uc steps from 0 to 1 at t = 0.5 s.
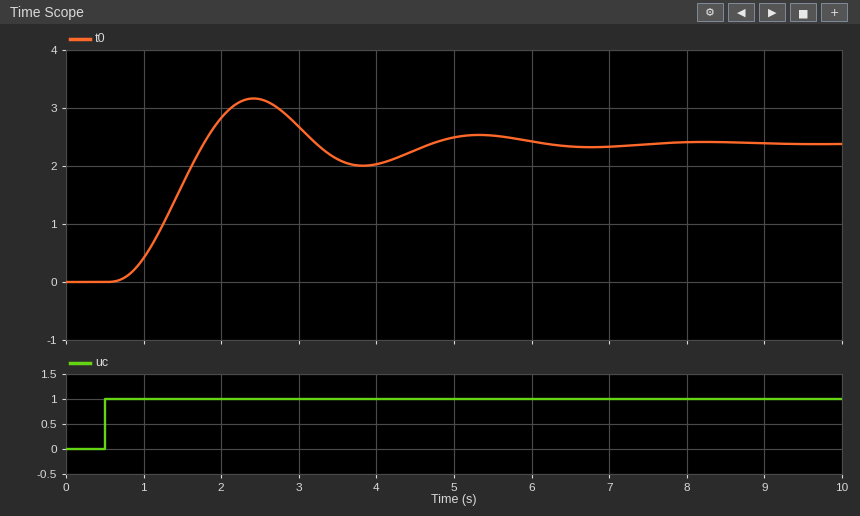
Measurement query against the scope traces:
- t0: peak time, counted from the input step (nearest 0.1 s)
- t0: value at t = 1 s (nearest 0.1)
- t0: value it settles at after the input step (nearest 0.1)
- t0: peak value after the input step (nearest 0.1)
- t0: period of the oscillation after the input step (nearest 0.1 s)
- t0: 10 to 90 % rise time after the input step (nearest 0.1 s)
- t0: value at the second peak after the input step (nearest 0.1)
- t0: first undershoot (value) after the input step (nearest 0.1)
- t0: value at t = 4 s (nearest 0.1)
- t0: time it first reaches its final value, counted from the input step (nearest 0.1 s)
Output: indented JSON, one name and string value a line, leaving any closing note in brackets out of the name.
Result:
{
  "t0: peak time, counted from the input step": "1.9 s",
  "t0: value at t = 1 s": "0.4",
  "t0: value it settles at after the input step": "2.4",
  "t0: peak value after the input step": "3.2",
  "t0: period of the oscillation after the input step": "2.9 s",
  "t0: 10 to 90 % rise time after the input step": "0.8 s",
  "t0: value at the second peak after the input step": "2.5",
  "t0: first undershoot (value) after the input step": "2.0",
  "t0: value at t = 4 s": "2.0",
  "t0: time it first reaches its final value, counted from the input step": "1.3 s"
}
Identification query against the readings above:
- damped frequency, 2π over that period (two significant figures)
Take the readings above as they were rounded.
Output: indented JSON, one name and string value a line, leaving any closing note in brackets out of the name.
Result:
{
  "damped frequency, 2π over that period": "2.2 rad/s"
}
